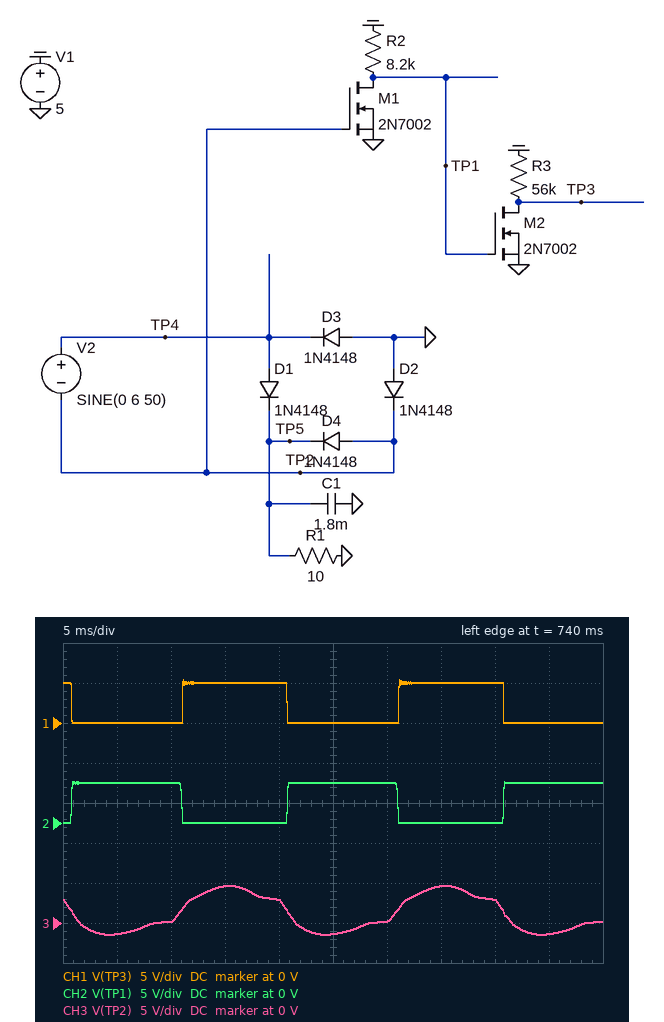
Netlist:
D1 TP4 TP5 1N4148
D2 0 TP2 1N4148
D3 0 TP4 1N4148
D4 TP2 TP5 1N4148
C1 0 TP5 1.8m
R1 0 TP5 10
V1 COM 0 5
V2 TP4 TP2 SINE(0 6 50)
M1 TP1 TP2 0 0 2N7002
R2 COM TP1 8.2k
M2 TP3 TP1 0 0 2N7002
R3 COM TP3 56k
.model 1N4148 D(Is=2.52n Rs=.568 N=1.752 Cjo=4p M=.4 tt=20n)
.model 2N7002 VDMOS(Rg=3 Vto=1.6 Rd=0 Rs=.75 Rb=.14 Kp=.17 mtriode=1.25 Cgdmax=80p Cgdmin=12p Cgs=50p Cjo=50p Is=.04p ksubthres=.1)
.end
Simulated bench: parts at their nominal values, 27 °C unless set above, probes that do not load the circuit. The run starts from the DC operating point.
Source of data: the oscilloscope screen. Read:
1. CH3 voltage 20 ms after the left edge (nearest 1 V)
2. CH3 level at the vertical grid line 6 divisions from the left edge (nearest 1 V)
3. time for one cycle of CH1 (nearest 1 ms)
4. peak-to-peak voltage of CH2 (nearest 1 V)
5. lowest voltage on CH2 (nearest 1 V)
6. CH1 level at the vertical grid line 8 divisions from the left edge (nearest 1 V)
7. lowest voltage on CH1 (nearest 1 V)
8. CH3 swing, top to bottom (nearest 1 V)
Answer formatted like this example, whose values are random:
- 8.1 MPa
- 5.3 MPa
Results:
- 3 V
- 0 V
- 20 ms
- 5 V
- 0 V
- 5 V
- 0 V
- 6 V
